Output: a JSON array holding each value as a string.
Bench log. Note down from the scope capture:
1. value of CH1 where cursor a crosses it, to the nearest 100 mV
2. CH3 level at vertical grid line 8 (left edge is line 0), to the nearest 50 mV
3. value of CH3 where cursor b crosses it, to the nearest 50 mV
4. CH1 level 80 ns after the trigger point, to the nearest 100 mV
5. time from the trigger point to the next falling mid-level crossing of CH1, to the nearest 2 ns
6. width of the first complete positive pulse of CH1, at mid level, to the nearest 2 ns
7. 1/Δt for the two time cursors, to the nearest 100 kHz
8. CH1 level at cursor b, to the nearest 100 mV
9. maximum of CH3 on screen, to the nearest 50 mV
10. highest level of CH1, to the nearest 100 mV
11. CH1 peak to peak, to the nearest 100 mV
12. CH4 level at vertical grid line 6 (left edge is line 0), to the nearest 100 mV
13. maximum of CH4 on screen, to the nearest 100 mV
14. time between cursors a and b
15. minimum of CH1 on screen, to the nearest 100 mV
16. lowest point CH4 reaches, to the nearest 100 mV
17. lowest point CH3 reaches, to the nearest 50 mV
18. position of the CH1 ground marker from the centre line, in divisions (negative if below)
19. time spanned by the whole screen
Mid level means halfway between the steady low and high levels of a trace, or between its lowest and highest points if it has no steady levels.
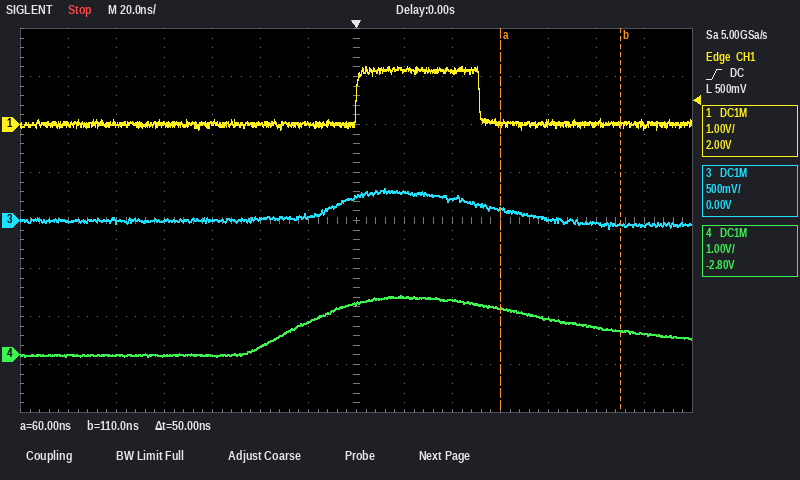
["0.0 V", "300 mV", "-50 mV", "0.0 V", "52 ns", "52 ns", "20.0 MHz", "0.0 V", "350 mV", "1.2 V", "1.3 V", "700 mV", "1.2 V", "50 ns", "-100 mV", "0.0 V", "-100 mV", "+2.0 div", "280 ns"]
